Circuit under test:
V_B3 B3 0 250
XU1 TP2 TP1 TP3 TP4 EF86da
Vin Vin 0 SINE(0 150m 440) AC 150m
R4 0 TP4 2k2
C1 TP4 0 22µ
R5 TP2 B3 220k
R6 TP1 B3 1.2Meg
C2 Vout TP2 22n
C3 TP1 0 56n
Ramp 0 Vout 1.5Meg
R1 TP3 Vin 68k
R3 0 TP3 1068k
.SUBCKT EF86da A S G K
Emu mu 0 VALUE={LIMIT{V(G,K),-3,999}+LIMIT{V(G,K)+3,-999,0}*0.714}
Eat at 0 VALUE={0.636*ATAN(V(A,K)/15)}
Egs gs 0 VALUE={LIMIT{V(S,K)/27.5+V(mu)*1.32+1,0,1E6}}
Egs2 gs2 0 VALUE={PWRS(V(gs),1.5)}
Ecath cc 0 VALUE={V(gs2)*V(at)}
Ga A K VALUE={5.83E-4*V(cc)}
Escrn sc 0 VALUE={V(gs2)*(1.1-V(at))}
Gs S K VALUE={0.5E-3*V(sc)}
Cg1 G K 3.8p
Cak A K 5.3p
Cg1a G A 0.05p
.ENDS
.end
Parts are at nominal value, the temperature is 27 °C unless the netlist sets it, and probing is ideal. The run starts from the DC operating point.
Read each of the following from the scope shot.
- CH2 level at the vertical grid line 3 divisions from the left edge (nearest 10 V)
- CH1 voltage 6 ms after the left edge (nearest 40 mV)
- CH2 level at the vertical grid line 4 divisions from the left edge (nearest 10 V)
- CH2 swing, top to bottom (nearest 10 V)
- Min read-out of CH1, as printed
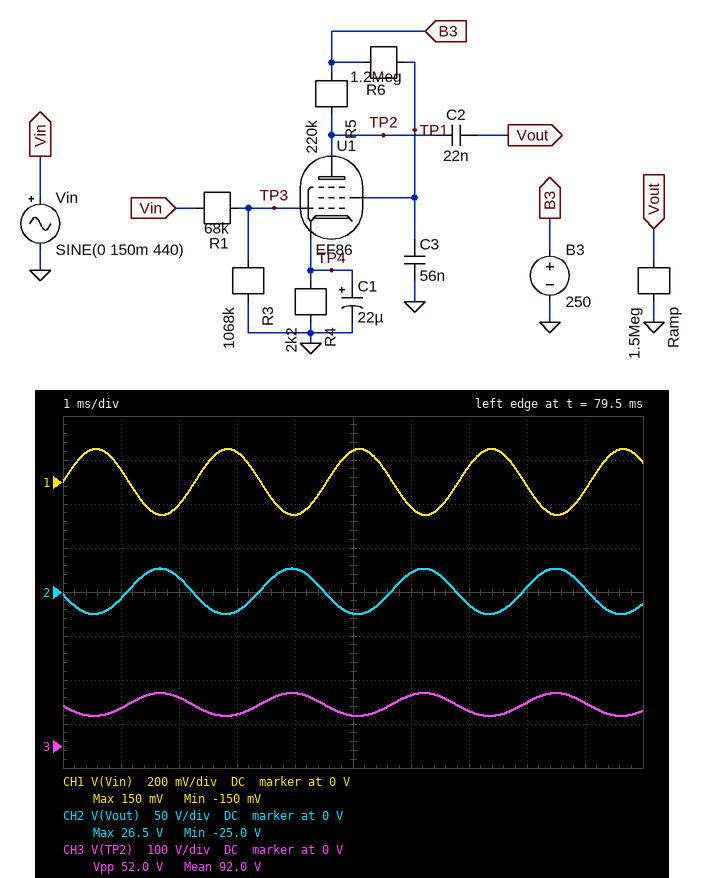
-20 V
-120 mV
30 V
50 V
-150 mV
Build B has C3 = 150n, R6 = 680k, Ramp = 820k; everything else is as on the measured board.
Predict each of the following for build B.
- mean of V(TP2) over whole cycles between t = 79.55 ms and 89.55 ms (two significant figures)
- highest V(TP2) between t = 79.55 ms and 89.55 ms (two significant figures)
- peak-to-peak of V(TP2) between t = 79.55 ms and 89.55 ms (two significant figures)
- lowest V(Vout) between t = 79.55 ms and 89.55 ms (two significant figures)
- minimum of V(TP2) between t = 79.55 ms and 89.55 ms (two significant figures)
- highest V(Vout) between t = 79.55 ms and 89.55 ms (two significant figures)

66 V
87 V
40 V
-19 V
47 V
21 V
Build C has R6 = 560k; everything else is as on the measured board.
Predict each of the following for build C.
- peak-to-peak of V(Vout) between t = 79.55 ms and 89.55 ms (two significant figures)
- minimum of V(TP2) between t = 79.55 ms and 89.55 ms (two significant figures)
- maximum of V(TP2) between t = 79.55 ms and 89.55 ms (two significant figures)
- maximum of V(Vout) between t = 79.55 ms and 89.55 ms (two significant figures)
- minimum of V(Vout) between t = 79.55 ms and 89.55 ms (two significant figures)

38 V
41 V
79 V
21 V
-17 V
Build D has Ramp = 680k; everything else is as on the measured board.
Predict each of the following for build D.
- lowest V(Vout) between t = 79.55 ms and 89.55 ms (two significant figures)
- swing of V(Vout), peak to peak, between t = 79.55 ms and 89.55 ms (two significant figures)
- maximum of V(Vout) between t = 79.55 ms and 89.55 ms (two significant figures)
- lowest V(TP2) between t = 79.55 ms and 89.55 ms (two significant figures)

-23 V
46 V
23 V
71 V
